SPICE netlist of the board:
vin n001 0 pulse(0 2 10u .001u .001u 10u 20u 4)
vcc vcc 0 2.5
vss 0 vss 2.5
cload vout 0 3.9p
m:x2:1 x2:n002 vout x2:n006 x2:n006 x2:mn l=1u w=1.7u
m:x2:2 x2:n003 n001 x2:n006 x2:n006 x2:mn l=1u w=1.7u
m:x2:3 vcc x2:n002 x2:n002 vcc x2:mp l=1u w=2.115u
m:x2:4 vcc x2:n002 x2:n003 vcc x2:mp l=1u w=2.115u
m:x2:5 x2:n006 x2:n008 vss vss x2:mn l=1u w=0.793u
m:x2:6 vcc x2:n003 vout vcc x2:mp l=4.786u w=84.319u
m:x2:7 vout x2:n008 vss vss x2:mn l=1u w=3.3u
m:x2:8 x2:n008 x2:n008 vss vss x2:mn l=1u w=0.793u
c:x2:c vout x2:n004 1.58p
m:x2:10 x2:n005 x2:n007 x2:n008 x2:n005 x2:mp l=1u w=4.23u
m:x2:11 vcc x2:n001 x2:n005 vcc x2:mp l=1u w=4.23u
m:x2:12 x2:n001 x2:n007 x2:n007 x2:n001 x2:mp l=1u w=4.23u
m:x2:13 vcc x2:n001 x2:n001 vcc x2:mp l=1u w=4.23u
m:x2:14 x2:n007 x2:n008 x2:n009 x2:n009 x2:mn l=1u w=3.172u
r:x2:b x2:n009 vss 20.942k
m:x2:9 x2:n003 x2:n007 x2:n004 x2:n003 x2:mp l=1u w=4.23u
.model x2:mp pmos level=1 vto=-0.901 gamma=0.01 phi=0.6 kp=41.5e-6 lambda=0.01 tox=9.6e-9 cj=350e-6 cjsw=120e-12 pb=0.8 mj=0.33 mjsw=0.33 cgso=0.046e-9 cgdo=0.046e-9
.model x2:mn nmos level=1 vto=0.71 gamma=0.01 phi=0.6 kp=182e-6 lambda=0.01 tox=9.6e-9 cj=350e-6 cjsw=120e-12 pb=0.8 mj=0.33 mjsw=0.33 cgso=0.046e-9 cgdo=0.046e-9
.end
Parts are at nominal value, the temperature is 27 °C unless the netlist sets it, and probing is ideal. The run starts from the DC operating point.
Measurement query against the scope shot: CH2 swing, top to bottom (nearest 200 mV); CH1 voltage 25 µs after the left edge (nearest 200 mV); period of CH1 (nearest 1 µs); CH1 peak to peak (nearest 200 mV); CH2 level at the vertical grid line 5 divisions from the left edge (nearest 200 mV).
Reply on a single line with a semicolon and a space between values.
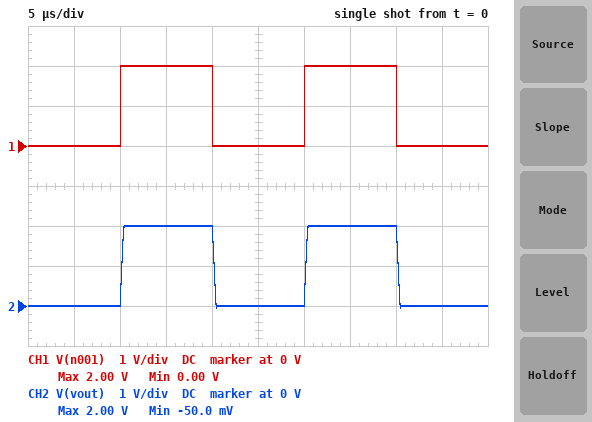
2.0 V; 0 V; 20 µs; 2.0 V; 0 V
